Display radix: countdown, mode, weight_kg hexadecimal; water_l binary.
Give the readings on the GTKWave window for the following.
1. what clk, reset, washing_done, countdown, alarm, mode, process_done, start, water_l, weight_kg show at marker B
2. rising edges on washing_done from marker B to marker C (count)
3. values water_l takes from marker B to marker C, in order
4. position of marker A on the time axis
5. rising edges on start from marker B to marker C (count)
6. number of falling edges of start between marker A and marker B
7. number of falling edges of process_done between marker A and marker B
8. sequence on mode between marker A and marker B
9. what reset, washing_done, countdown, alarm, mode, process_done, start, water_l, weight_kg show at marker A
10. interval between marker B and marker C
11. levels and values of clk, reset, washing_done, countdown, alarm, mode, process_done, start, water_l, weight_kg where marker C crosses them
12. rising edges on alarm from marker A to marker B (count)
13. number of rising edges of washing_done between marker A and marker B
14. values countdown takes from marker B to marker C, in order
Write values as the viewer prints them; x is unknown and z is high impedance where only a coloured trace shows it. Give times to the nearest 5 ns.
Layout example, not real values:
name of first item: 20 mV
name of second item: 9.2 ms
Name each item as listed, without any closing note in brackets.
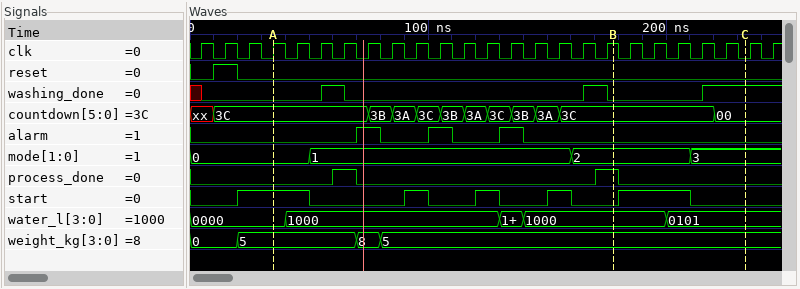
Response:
what clk, reset, washing_done, countdown, alarm, mode, process_done, start, water_l, weight_kg show at marker B: clk=1, reset=0, washing_done=0, countdown=3C, alarm=0, mode=2, process_done=1, start=0, water_l=1000, weight_kg=5
rising edges on washing_done from marker B to marker C: 1
values water_l takes from marker B to marker C, in order: 1000, 0101
position of marker A on the time axis: 35 ns
rising edges on start from marker B to marker C: 1
number of falling edges of start between marker A and marker B: 4
number of falling edges of process_done between marker A and marker B: 1
sequence on mode between marker A and marker B: 0, 1, 2
what reset, washing_done, countdown, alarm, mode, process_done, start, water_l, weight_kg show at marker A: reset=0, washing_done=0, countdown=3C, alarm=0, mode=0, process_done=0, start=1, water_l=0000, weight_kg=5
interval between marker B and marker C: 55 ns
levels and values of clk, reset, washing_done, countdown, alarm, mode, process_done, start, water_l, weight_kg where marker C crosses them: clk=0, reset=0, washing_done=1, countdown=00, alarm=0, mode=3, process_done=0, start=0, water_l=0101, weight_kg=5
rising edges on alarm from marker A to marker B: 3
number of rising edges of washing_done between marker A and marker B: 2
values countdown takes from marker B to marker C, in order: 3C, 00
